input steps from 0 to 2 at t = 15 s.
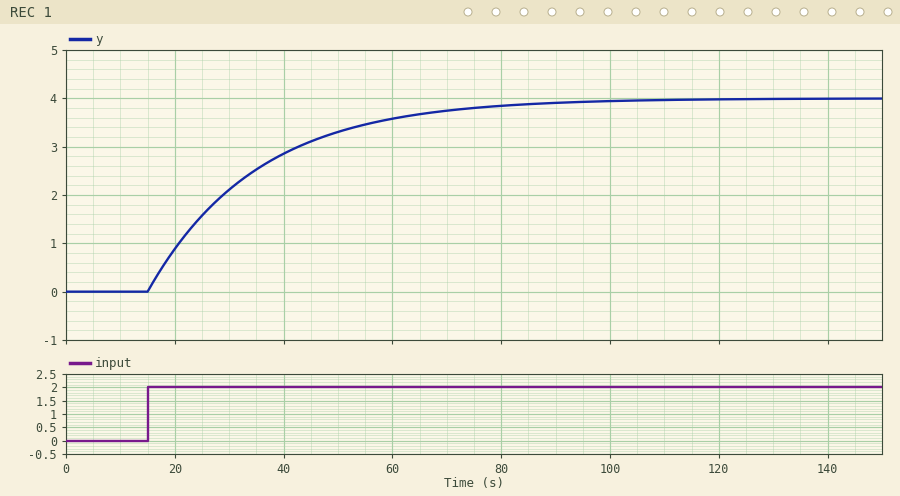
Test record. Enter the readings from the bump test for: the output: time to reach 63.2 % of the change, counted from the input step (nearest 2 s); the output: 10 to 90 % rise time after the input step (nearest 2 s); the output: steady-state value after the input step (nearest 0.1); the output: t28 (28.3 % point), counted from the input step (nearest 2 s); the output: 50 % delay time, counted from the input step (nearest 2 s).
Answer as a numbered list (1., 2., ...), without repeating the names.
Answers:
1. 20 s
2. 44 s
3. 4.0
4. 6 s
5. 14 s
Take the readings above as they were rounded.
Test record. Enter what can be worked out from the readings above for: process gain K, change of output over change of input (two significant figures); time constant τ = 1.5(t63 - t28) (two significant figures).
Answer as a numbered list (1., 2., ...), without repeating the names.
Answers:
1. 2.0
2. 21 s
